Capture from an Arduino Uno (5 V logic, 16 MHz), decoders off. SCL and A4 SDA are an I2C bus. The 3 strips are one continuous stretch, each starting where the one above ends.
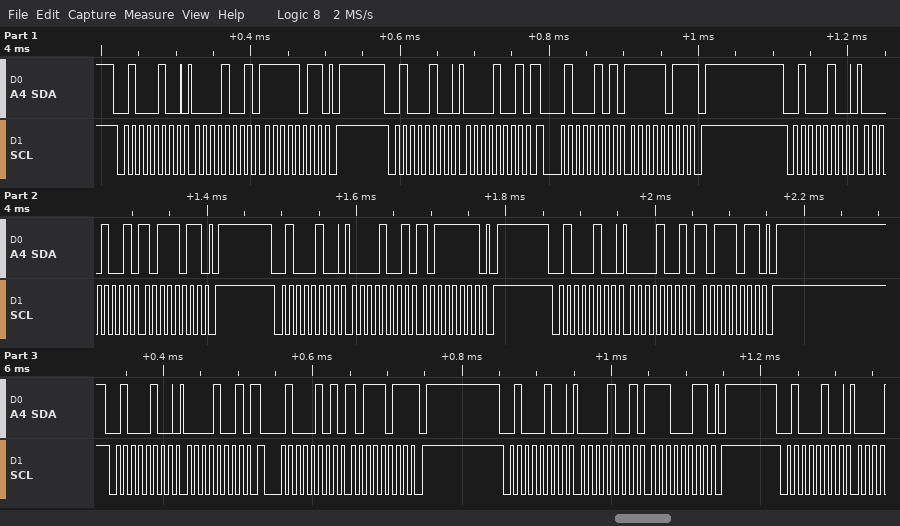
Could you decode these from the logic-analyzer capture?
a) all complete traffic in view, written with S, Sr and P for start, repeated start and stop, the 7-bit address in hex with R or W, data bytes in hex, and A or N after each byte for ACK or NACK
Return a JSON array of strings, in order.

["S 22W A 09 A FB A P S 22W A 09 A Sr 22R A FB N P S 22W A 09 A BB A P S 22W A 09 A BF A P S 22W A 09 A BB A P S 22W A 09 A Sr 22R A BB N P S 22W A 09 A E3 A P S 22W A"]
